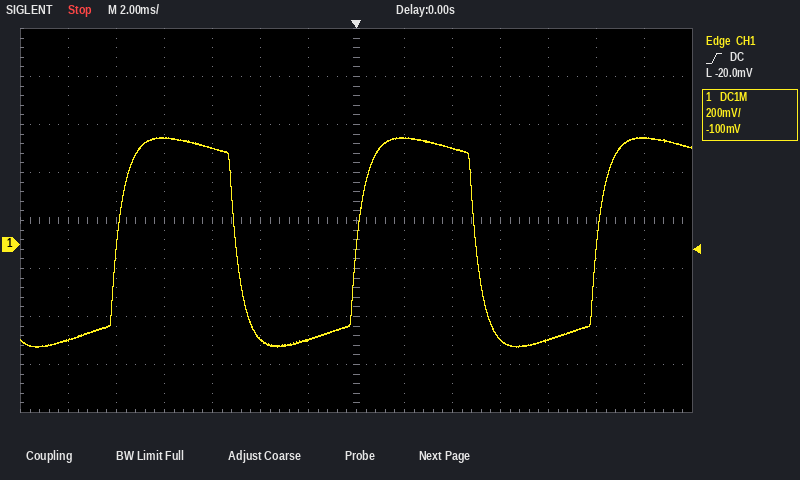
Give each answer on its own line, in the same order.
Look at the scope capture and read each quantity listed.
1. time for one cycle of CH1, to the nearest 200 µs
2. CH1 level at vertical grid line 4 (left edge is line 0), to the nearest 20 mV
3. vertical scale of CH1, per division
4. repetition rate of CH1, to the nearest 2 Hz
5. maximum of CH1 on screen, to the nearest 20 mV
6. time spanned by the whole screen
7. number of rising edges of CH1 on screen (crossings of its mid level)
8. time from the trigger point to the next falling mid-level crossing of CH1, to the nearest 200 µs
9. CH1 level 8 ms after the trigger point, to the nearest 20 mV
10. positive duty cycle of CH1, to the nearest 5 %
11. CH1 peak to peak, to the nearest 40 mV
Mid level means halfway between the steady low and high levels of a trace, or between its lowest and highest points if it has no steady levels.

10.0 ms
400 mV
200 mV
100 Hz
440 mV
28 ms
3
5.0 ms
-400 mV
50 %
880 mV
